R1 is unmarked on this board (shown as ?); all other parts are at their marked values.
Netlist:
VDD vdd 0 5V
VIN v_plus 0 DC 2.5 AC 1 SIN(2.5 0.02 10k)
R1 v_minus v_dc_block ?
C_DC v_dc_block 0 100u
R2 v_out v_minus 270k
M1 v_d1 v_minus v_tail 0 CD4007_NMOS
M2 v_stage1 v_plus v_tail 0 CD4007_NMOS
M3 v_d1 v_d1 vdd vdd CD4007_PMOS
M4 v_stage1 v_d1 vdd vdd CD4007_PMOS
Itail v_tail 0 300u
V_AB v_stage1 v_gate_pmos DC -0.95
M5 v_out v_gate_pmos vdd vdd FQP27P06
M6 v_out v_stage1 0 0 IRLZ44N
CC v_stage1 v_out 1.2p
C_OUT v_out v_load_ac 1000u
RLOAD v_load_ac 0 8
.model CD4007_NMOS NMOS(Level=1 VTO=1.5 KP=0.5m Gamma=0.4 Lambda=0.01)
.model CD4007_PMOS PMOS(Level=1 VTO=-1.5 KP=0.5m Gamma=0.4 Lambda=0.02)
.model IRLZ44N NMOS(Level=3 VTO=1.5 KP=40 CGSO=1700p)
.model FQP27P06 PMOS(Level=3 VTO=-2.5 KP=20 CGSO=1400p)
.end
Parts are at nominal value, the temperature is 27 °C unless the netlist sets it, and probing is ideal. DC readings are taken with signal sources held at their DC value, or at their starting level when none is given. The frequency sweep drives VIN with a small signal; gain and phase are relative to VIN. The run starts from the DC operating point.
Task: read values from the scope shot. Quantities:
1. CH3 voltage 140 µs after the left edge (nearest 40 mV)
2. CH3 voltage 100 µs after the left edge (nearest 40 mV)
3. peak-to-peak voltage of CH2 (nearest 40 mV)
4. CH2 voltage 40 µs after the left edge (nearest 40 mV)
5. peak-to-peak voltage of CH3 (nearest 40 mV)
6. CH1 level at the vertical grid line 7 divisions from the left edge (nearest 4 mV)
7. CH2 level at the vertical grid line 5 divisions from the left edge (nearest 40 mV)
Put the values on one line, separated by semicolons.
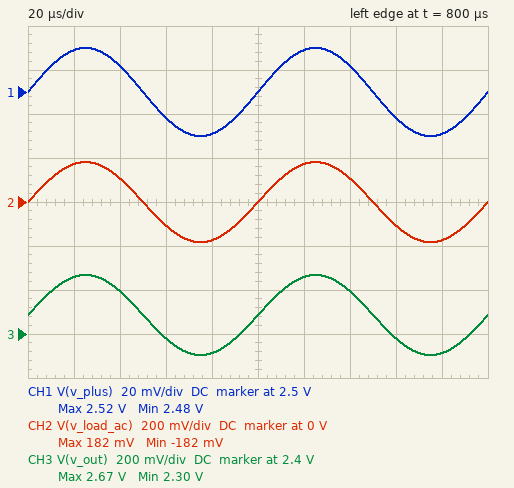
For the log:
2.60 V; 2.48 V; 360 mV; 120 mV; 360 mV; 2.512 V; 0 V
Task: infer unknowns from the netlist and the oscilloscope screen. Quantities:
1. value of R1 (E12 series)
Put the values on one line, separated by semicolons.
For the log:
33 kΩ
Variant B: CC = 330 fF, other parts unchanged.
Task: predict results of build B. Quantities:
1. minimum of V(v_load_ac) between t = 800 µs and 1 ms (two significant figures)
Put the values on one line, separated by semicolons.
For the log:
-180 mV
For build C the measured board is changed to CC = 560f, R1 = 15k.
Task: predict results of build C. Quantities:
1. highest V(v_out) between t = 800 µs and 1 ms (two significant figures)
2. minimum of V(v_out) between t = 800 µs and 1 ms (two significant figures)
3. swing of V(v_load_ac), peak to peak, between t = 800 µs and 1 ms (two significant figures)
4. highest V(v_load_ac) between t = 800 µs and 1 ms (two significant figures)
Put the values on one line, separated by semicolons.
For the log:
2.9 V; 2.1 V; 750 mV; 370 mV
